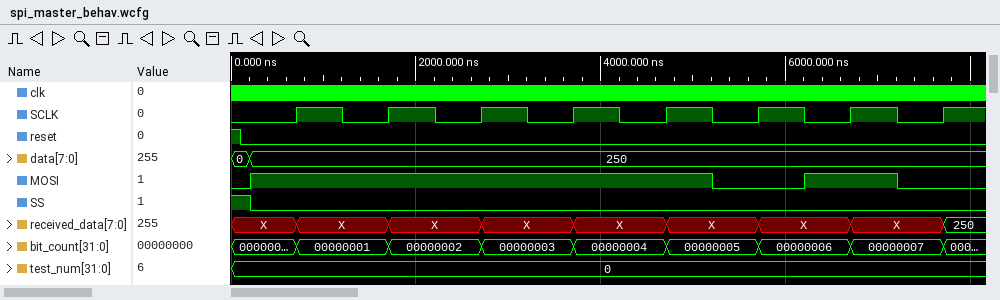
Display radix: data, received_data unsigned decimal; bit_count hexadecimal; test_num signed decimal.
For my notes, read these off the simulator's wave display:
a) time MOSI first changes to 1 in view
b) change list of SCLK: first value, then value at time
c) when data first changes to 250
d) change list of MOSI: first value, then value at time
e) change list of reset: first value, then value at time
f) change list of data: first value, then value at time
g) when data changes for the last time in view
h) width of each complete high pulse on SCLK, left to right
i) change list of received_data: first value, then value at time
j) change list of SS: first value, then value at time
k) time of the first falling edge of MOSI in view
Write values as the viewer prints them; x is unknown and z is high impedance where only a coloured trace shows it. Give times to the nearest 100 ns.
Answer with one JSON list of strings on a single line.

["200 ns", "0, 1 at 700 ns, 0 at 1200 ns, 1 at 1700 ns, 0 at 2200 ns, 1 at 2700 ns, 0 at 3200 ns, 1 at 3700 ns, 0 at 4200 ns, 1 at 4700 ns, 0 at 5200 ns, 1 at 5700 ns, 0 at 6200 ns, 1 at 6700 ns, 0 at 7200 ns, 1 at 7700 ns", "200 ns", "0, 1 at 200 ns, 0 at 5200 ns, 1 at 6200 ns, 0 at 7200 ns", "1, 0 at 100 ns", "0, 250 at 200 ns", "200 ns", "500 ns, 500 ns, 500 ns, 500 ns, 500 ns, 500 ns, 500 ns", "X, X at 700 ns, X at 1700 ns, X at 2700 ns, X at 3700 ns, X at 4700 ns, X at 5700 ns, X at 6700 ns, 250 at 7700 ns", "1, 0 at 200 ns", "5200 ns"]
